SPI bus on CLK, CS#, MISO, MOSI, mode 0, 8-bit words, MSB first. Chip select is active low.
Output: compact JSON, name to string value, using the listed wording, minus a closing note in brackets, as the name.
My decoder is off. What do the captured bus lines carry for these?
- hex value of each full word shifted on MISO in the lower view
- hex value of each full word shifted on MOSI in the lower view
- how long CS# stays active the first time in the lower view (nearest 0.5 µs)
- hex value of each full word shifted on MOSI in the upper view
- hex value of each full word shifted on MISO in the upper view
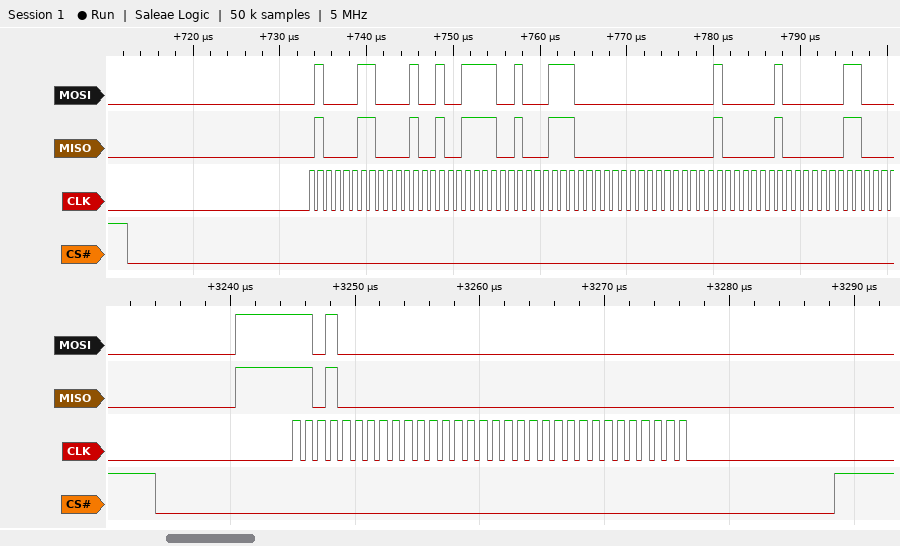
{"hex value of each full word shifted on MISO in the lower view": "D0, 00, 00, 00", "hex value of each full word shifted on MOSI in the lower view": "D0, 00, 00, 00", "how long CS# stays active the first time in the lower view": "54.5 µs", "hex value of each full word shifted on MOSI in the upper view": "43, 09, 3C, 8E, 00, 01, 02, 03", "hex value of each full word shifted on MISO in the upper view": "43, 09, 3C, 8E, 00, 01, 02, 03"}
